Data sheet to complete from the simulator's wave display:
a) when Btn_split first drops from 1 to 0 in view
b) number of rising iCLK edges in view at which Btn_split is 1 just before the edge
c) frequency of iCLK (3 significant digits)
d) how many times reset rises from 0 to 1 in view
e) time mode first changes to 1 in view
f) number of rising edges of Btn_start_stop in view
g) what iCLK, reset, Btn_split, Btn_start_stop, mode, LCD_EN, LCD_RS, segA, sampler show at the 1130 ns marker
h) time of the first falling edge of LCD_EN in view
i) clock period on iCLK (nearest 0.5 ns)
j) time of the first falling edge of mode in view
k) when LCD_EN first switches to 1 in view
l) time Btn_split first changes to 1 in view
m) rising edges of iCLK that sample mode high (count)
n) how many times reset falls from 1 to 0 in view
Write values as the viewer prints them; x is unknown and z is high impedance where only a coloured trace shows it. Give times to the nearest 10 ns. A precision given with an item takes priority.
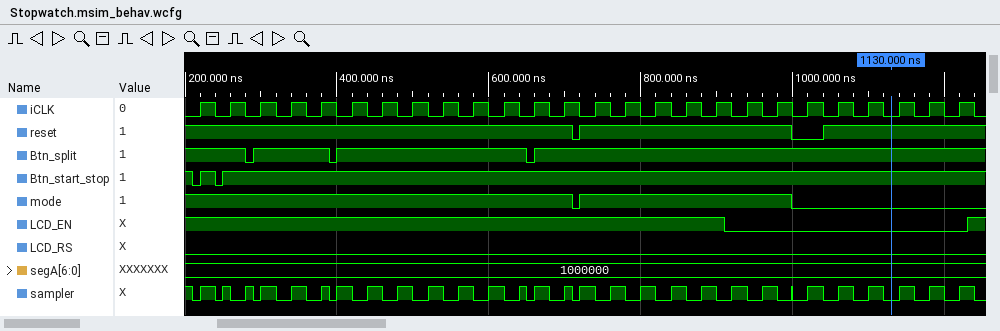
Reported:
280 ns
25
25.0 MHz
2
720 ns
2
iCLK=0, reset=1, Btn_split=1, Btn_start_stop=1, mode=0, LCD_EN=0, LCD_RS=0, segA=1000000, sampler=0
910 ns
40 ns
710 ns
1230 ns
290 ns
20
2
